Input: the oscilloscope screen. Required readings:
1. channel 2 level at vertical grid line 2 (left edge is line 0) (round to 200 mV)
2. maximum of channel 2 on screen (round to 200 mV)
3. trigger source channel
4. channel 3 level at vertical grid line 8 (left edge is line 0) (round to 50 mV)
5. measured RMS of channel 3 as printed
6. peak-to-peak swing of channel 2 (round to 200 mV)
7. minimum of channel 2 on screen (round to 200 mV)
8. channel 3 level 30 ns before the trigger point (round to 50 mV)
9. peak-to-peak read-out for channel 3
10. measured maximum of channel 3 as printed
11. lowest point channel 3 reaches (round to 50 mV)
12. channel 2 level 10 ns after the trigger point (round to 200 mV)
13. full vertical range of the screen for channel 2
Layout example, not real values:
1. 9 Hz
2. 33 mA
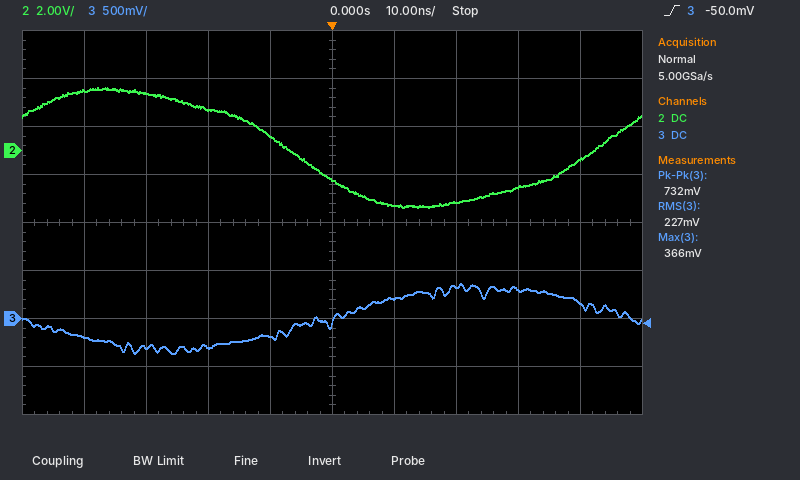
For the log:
1. 2.4 V
2. 2.6 V
3. channel 3
4. 300 mV
5. 227 mV
6. 5.0 V
7. -2.4 V
8. -300 mV
9. 732 mV
10. 366 mV
11. -350 mV
12. -2.2 V
13. 16 V
